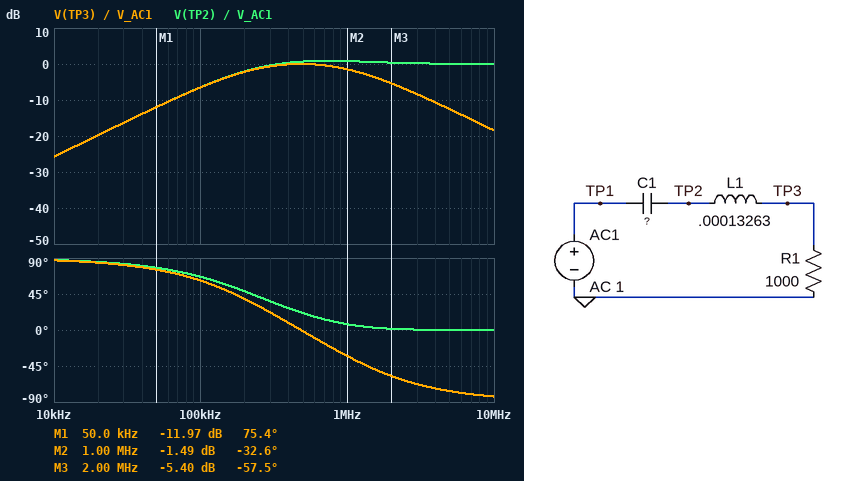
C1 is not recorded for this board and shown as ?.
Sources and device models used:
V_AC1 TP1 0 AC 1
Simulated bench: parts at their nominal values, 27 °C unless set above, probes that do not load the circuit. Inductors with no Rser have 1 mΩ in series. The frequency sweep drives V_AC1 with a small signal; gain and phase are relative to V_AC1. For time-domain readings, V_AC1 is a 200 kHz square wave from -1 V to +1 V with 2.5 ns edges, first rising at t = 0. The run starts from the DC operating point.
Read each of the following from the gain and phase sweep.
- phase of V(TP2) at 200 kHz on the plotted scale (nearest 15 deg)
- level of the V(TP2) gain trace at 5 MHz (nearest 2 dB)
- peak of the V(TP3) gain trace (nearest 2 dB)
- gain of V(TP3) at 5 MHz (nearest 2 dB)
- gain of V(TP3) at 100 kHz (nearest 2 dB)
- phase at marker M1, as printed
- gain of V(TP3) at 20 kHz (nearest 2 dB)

45 deg
0 dB
0 dB
-12 dB
-6 dB
75.4 deg
-20 dB
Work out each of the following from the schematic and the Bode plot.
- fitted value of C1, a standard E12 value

820 pF
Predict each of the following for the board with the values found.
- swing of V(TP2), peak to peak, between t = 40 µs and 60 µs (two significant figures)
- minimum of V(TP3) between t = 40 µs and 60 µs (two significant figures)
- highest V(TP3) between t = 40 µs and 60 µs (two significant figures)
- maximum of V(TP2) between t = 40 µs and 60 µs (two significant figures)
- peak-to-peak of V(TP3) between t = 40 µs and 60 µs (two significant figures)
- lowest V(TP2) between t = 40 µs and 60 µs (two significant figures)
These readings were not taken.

3.9 V
-1.5 V
1.5 V
1.9 V
3.1 V
-1.9 V
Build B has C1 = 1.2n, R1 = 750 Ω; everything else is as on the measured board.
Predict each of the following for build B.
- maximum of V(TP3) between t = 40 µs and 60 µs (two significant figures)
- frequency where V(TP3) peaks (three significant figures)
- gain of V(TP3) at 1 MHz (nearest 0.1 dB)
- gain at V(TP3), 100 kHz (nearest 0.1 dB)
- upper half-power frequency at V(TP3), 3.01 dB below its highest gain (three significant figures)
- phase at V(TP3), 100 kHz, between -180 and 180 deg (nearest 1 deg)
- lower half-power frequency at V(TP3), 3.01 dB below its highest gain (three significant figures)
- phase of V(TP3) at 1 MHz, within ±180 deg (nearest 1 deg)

1.5 V
399 kHz
-2.7 dB
-5.7 dB
1.05 MHz
59 deg
151 kHz
-43 deg
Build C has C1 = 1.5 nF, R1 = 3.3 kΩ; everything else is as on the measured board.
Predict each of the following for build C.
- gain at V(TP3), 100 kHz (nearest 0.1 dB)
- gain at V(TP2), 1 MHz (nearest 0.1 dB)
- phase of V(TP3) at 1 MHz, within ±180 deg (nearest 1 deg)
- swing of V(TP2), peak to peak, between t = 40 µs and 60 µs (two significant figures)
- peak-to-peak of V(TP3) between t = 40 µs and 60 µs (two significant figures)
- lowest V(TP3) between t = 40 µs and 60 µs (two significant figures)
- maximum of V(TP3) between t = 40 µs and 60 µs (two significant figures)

-0.4 dB
0.1 dB
-12 deg
2.5 V
2.4 V
-1.2 V
1.2 V
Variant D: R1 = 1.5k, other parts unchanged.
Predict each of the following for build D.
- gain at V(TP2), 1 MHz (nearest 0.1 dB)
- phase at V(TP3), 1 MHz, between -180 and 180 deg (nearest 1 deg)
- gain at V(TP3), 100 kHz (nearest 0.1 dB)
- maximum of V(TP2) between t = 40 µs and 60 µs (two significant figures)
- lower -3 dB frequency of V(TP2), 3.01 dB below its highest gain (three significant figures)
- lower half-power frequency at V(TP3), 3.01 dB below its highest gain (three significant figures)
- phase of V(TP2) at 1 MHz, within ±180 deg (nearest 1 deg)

0.4 dB
-23 deg
-4.0 dB
1.8 V
133 kHz
121 kHz
6 deg
